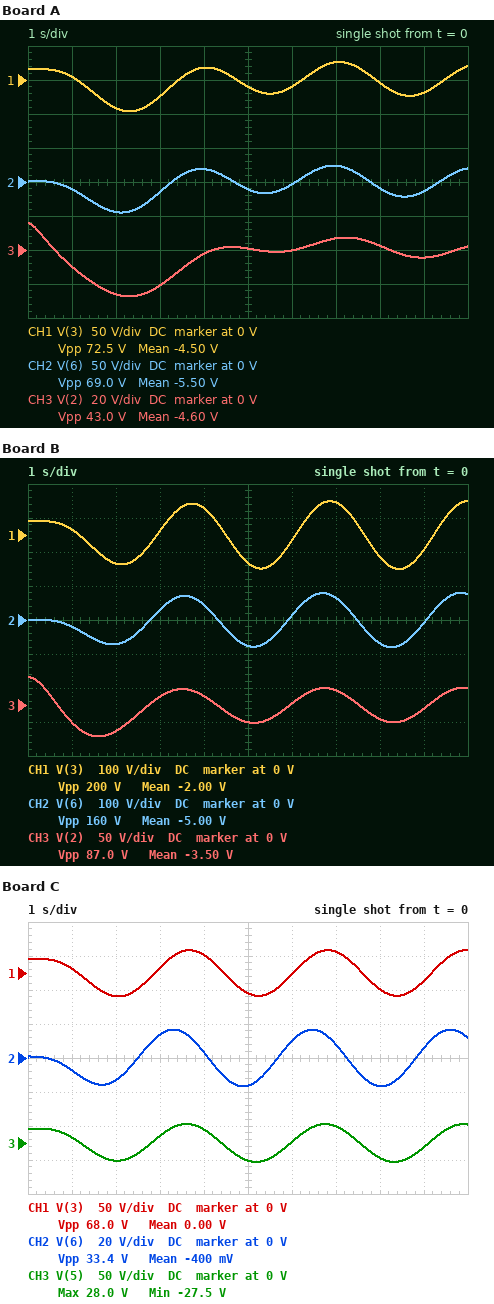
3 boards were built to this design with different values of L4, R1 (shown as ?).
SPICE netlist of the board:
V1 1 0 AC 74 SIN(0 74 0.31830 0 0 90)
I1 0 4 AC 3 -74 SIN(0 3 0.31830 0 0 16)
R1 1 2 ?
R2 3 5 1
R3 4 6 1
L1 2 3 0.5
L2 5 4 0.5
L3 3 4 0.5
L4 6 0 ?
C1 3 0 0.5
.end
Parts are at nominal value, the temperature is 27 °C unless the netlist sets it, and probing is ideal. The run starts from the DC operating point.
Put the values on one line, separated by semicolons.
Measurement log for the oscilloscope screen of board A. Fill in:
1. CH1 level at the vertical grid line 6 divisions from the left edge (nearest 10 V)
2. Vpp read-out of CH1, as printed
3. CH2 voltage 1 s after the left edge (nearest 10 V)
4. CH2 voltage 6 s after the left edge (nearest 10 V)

-10 V; 72.5 V; -10 V; 0 V
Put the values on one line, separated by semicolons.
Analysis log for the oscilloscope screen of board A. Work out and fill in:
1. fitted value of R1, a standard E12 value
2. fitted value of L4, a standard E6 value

3.9 Ω; 3.3 H
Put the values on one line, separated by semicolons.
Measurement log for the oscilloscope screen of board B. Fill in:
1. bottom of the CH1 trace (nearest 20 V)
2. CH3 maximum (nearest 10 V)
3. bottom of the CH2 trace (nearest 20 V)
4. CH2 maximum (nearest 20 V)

-100 V; 40 V; -80 V; 80 V
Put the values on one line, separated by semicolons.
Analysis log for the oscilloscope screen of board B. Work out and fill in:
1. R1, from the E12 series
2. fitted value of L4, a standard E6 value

0.82 Ω; 1.5 H
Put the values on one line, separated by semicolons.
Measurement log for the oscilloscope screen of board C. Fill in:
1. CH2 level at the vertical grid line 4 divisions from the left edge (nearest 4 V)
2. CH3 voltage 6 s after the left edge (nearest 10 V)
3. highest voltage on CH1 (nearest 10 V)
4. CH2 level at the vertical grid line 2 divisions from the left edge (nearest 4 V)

4 V; 0 V; 30 V; -12 V
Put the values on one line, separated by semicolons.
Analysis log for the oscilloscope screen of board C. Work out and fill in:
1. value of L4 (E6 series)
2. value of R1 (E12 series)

470 mH; 2.7 Ω
